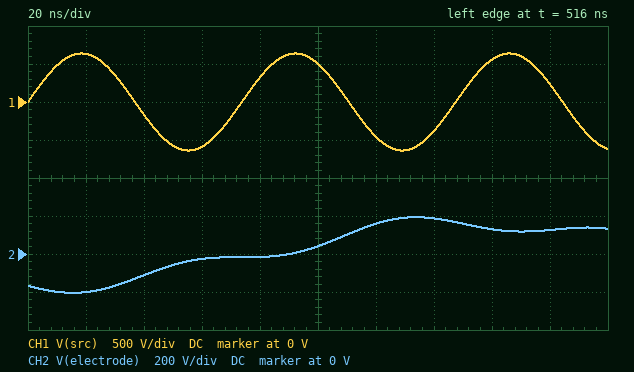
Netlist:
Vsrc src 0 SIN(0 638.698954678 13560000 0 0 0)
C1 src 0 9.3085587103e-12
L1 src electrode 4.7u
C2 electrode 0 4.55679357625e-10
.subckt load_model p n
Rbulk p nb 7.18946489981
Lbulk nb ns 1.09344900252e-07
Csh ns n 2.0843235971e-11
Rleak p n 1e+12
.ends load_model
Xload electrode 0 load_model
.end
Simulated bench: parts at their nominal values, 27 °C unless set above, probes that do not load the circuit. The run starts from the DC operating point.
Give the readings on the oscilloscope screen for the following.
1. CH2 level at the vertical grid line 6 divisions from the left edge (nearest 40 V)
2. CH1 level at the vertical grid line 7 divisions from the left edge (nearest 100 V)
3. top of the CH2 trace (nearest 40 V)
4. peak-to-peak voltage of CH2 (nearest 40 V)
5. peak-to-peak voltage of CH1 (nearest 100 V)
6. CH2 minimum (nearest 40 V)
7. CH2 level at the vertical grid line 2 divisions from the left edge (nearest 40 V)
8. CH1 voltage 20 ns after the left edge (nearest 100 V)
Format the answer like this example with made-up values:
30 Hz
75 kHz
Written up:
160 V
-400 V
200 V
400 V
1.3 kV
-200 V
-120 V
600 V
